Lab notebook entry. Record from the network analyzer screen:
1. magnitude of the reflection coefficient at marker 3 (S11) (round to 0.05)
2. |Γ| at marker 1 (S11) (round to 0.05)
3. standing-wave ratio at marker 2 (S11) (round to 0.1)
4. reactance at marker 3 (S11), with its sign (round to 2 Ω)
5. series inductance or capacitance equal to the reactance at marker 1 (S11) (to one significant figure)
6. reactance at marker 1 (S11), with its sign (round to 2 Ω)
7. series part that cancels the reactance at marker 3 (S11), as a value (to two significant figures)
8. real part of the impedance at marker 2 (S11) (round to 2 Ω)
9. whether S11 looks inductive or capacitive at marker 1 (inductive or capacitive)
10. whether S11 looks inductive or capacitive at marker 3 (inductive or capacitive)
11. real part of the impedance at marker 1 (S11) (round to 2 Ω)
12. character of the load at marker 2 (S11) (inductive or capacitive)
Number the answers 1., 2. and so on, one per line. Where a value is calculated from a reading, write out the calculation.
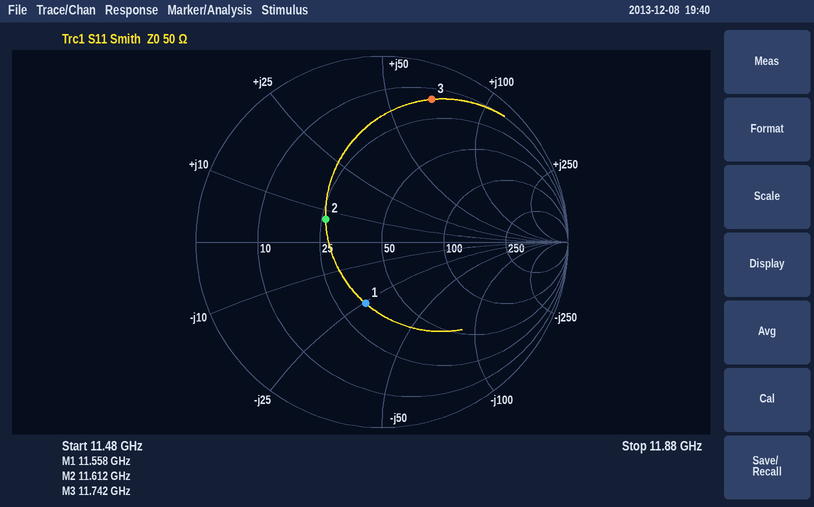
1. 0.80
2. 0.35
3. 2.0
4. +68 Ω
5. C = 1/(2π × 11.558 GHz × 26 Ω) ≈ 530 fF, so 500 fF to one significant figure
6. -26 Ω
7. C = 1/(2π × 11.742 GHz × 68 Ω) ≈ 199 fF, so 200 fF to two significant figures
8. 26 Ω
9. capacitive
10. inductive
11. 34 Ω
12. inductive
